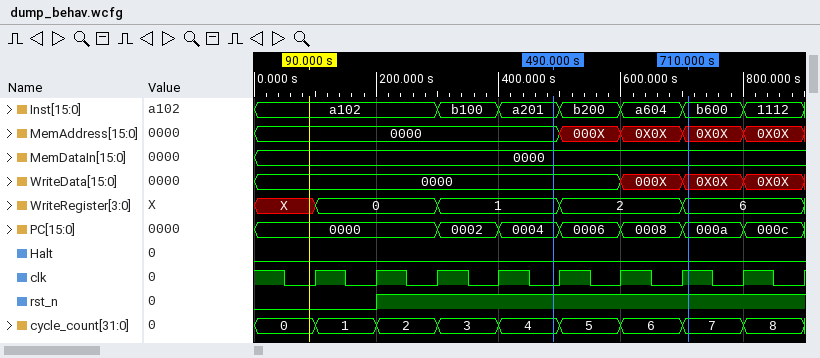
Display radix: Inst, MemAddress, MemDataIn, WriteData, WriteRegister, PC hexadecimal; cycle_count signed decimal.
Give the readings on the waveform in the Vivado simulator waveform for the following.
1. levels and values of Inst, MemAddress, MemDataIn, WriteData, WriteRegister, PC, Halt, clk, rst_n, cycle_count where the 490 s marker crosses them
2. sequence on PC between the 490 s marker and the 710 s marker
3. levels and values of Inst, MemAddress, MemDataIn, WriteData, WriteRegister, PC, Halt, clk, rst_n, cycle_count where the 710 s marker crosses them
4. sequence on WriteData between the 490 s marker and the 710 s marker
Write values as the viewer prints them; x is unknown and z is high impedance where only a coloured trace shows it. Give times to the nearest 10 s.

Inst=a201, MemAddress=0000, MemDataIn=0000, WriteData=0000, WriteRegister=1, PC=0004, Halt=0, clk=0, rst_n=1, cycle_count=4
0004, 0006, 0008, 000a
Inst=b600, MemAddress=0X0X, MemDataIn=0000, WriteData=0X0X, WriteRegister=6, PC=000a, Halt=0, clk=1, rst_n=1, cycle_count=7
0000, 000X, 0X0X
